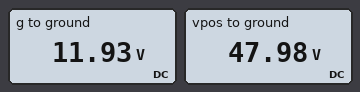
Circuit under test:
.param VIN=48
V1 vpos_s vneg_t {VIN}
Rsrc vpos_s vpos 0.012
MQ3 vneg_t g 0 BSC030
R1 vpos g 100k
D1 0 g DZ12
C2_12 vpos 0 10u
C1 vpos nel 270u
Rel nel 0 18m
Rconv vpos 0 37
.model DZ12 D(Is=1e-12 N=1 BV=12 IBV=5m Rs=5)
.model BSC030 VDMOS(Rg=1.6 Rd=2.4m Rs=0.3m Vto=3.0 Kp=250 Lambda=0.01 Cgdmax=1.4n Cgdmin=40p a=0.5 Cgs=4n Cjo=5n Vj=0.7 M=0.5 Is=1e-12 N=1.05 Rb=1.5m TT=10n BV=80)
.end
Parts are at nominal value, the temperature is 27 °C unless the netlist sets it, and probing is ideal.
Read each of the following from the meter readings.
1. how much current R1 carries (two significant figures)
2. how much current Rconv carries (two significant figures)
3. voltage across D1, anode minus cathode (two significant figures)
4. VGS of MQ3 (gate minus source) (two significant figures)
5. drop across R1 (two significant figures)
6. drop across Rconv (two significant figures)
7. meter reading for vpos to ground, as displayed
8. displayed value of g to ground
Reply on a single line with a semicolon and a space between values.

360 µA; 1.3 A; -12 V; 12 V; 36 V; 48 V; 47.98 V; 11.93 V
